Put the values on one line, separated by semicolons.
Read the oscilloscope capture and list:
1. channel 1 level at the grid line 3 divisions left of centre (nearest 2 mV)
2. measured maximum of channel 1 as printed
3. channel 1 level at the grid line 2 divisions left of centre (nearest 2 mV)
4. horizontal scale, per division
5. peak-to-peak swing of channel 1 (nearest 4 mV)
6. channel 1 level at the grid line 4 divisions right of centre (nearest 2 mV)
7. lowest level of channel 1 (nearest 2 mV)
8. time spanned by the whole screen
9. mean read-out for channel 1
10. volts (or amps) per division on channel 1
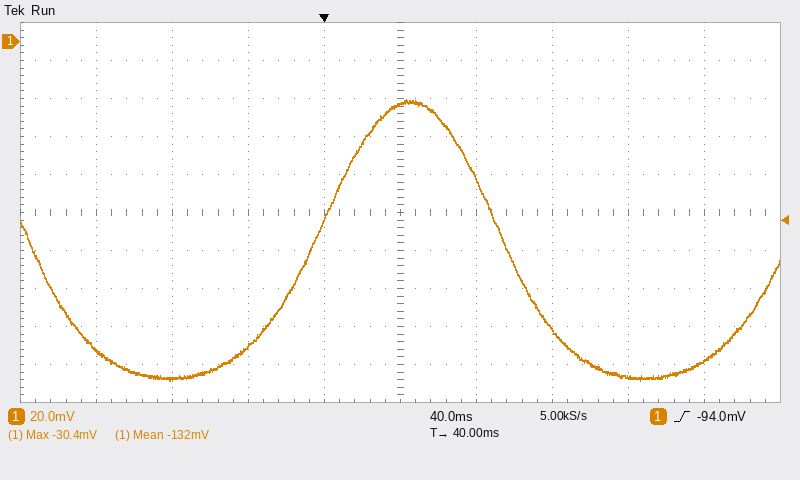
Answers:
-178 mV; -30.4 mV; -160 mV; 40 ms; 148 mV; -168 mV; -178 mV; 400 ms; -132 mV; 20 mV
